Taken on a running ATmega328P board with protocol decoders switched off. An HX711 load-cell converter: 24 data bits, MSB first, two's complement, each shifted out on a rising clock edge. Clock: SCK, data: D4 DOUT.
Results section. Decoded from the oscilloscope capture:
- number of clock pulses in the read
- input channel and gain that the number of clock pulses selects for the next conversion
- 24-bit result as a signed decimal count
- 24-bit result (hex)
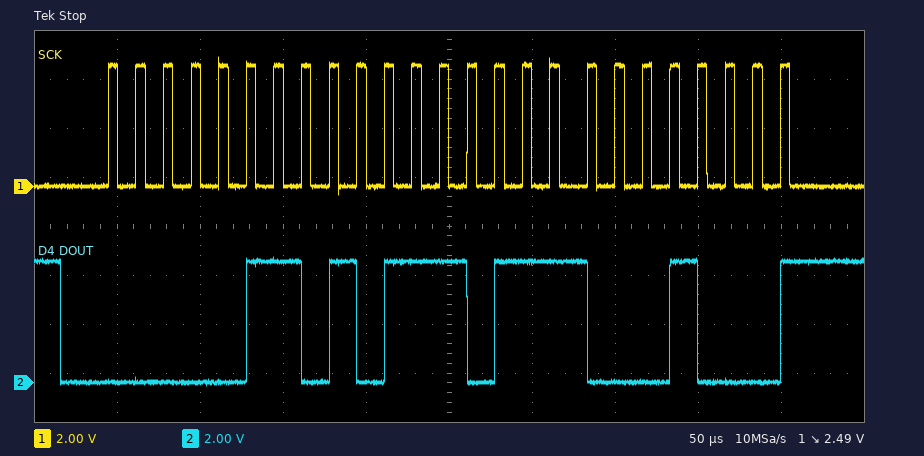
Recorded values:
25
channel A, gain 128
441224
0x06BB88
